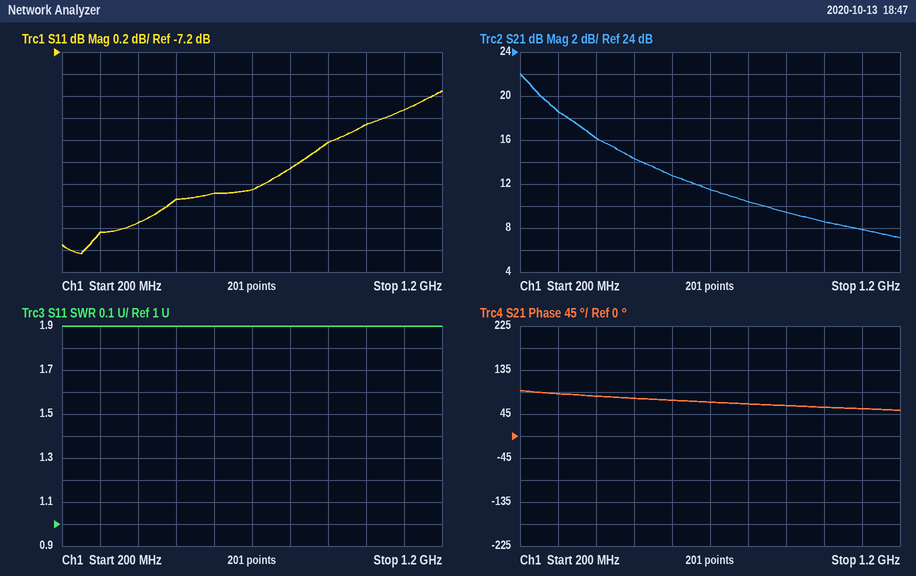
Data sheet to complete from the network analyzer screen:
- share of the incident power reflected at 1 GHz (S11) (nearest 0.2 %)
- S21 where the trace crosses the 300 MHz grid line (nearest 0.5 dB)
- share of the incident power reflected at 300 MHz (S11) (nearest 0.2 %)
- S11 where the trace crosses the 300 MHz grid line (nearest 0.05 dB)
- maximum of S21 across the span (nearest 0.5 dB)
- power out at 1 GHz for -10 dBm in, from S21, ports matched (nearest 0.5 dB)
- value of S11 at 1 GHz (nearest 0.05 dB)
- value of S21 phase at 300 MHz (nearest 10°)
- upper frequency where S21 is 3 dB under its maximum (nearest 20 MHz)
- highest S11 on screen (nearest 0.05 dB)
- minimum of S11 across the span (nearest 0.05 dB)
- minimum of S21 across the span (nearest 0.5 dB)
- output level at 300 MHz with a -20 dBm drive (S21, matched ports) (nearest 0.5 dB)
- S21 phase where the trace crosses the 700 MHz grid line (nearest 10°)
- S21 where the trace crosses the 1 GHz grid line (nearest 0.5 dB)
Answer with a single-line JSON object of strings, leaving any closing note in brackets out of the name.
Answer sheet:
{"share of the incident power reflected at 1 GHz (S11)": "16.4 %", "S21 where the trace crosses the 300 MHz grid line": "18.5 dB", "share of the incident power reflected at 300 MHz (S11)": "13.0 %", "S11 where the trace crosses the 300 MHz grid line": "-8.85 dB", "maximum of S21 across the span": "22.0 dB", "power out at 1 GHz for -10 dBm in, from S21, ports matched": "-1.5 dBm", "value of S11 at 1 GHz": "-7.85 dB", "value of S21 phase at 300 MHz": "90°", "upper frequency where S21 is 3 dB under its maximum": "280 MHz", "highest S11 on screen": "-7.55 dB", "minimum of S11 across the span": "-9.05 dB", "minimum of S21 across the span": "7.0 dB", "output level at 300 MHz with a -20 dBm drive (S21, matched ports)": "-1.5 dBm", "S21 phase where the trace crosses the 700 MHz grid line": "70°", "S21 where the trace crosses the 1 GHz grid line": "8.5 dB"}
